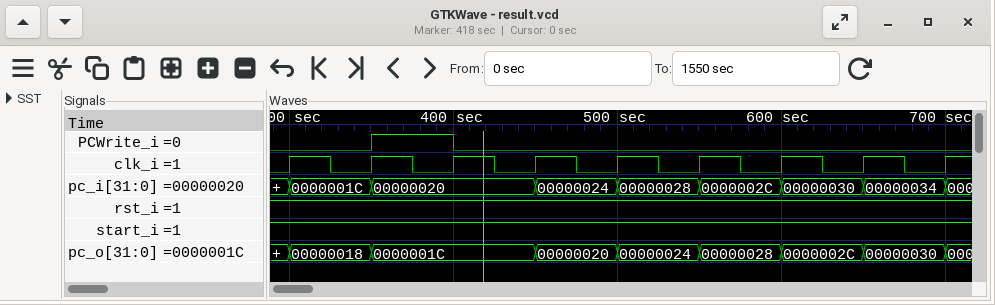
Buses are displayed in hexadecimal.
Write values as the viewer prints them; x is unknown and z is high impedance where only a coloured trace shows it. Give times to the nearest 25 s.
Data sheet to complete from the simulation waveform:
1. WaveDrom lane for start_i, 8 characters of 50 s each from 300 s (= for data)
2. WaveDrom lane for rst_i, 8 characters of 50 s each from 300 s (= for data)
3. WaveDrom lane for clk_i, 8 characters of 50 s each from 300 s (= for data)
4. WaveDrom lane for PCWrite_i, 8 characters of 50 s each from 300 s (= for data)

{name: 'start_i', wave: '1.......'}
{name: 'rst_i', wave: '1.......'}
{name: 'clk_i', wave: 'p.......'}
{name: 'PCWrite_i', wave: '010.....'}
